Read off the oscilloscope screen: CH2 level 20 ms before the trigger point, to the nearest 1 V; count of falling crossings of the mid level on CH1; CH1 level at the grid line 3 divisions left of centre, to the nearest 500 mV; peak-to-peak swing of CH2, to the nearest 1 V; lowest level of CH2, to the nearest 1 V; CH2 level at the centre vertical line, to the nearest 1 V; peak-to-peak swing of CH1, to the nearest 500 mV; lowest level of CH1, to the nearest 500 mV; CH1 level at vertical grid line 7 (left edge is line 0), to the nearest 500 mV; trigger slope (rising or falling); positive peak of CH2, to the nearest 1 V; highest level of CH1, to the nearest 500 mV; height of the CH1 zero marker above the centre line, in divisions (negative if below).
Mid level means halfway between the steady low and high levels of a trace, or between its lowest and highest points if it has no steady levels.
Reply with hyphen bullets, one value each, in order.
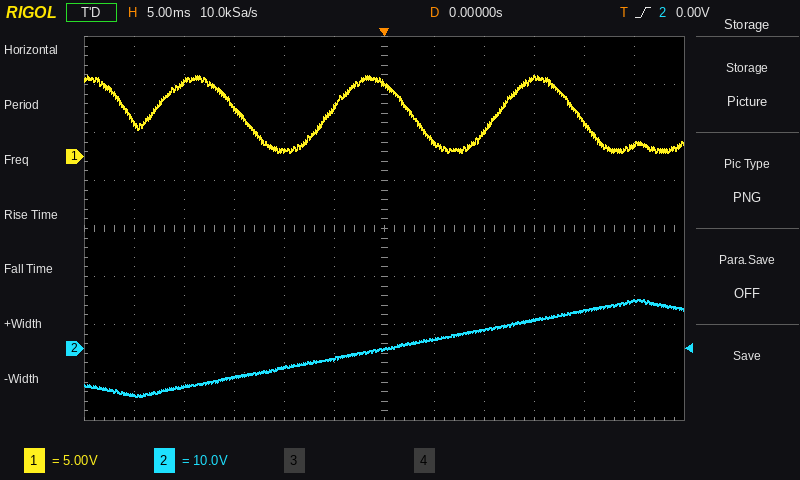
- -8 V
- 4
- 5.0 V
- 20 V
- -10 V
- 0 V
- 8.0 V
- 500 mV
- 1.5 V
- rising
- 10 V
- 8.5 V
- +1.5 div
